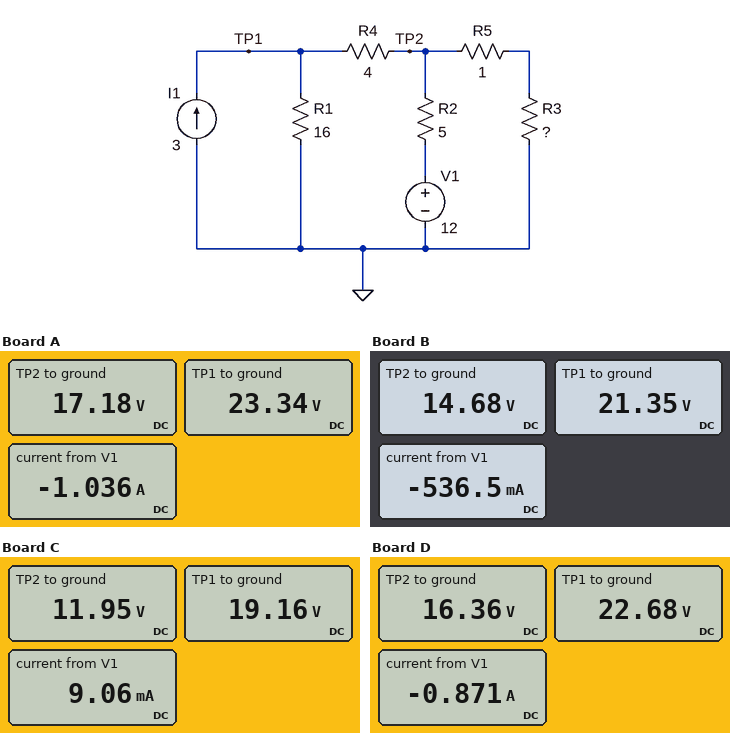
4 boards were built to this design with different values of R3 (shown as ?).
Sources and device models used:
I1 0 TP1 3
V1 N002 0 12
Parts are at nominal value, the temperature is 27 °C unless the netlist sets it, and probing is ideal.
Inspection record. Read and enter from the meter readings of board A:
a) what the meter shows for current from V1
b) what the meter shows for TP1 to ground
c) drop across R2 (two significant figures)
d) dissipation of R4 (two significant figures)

-1.036 A
23.34 V
5.2 V
9.5 W
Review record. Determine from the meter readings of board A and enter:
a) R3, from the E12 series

33 Ω
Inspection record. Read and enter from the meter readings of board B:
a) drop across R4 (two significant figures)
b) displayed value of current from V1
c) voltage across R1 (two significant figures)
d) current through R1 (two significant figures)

6.7 V
-536.5 mA
21 V
1.3 A
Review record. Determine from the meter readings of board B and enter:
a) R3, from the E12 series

12 Ω
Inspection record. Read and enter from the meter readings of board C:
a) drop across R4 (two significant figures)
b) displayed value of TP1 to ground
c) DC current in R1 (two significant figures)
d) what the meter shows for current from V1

7.2 V
19.16 V
1.2 A
9.06 mA
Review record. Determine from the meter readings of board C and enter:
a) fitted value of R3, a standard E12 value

5.6 Ω
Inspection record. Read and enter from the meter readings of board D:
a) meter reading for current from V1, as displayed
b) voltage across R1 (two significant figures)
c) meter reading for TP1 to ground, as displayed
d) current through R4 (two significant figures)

-0.871 A
23 V
22.68 V
1.6 A
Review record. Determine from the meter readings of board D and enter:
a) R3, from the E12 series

22 Ω
